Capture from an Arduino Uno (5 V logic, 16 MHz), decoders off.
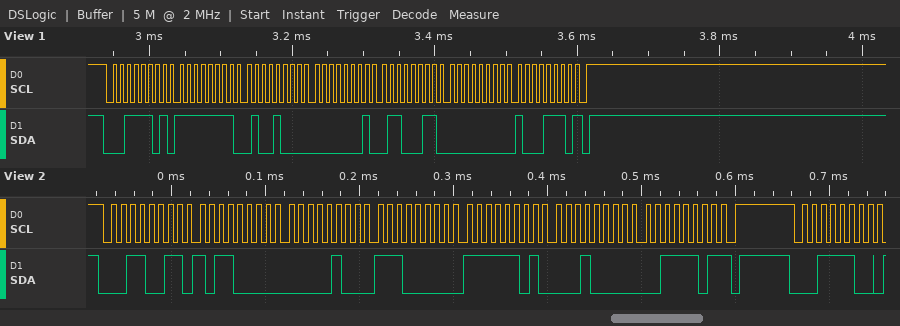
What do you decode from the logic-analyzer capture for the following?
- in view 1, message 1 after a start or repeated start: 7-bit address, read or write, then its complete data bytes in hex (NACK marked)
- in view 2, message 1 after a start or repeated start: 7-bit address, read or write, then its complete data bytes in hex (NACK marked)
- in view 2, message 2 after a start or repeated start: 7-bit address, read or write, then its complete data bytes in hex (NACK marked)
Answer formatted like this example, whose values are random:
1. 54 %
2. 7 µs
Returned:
1. 0x1E read: FF 48 01 63 00 8E NACK
2. 0x19 read: B0 04 E0 FD 10 3D NACK
3. 0x1E write
